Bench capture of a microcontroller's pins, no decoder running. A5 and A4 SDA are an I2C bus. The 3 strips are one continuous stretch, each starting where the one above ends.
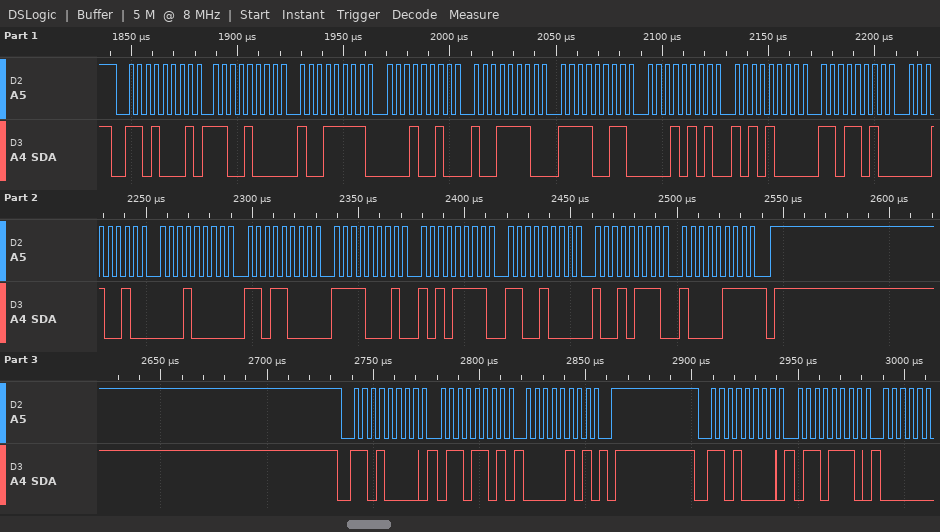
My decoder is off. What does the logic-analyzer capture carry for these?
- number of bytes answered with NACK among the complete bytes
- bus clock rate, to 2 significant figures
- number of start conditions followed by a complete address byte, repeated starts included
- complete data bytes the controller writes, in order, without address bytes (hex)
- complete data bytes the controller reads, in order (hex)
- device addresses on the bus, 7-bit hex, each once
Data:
1
250 kHz
3
6D 05 6E
C8 9F 12 9E F3 15 A8 DA 12 10 D8 F1 AF C8 97 87
0x68
